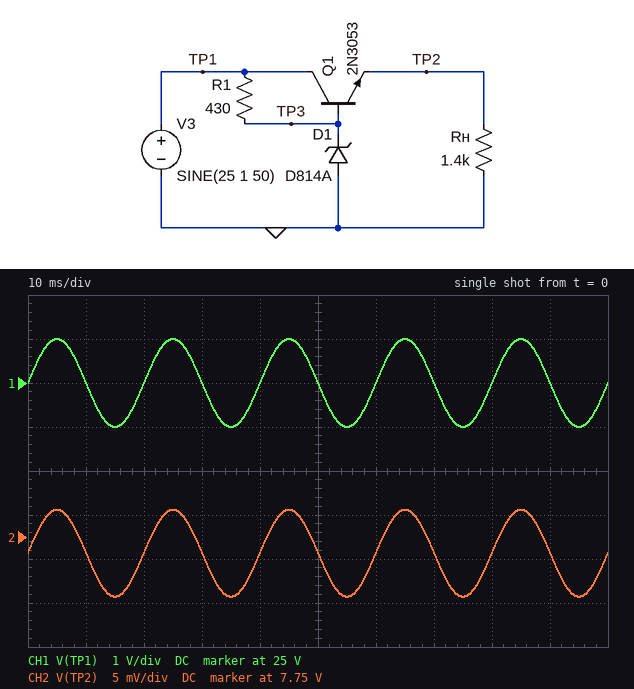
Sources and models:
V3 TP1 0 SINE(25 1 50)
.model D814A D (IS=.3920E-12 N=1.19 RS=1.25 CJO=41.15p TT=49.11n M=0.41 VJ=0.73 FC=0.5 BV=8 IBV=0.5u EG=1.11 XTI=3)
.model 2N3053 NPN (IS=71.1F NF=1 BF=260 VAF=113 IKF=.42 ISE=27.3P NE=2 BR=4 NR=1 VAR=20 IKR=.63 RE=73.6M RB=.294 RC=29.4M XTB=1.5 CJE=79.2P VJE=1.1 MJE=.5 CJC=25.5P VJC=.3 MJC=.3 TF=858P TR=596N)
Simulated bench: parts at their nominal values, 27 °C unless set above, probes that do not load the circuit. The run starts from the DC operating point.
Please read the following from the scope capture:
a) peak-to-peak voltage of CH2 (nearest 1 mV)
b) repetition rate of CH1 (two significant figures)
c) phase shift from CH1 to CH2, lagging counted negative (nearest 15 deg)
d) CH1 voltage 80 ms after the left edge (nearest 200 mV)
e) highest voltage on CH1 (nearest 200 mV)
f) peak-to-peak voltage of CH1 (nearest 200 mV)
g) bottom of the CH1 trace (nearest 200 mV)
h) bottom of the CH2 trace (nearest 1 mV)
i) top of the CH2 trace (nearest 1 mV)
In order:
10 mV
50 Hz
0 deg
25.0 V
26.0 V
2.0 V
24.0 V
7.743 V
7.753 V
